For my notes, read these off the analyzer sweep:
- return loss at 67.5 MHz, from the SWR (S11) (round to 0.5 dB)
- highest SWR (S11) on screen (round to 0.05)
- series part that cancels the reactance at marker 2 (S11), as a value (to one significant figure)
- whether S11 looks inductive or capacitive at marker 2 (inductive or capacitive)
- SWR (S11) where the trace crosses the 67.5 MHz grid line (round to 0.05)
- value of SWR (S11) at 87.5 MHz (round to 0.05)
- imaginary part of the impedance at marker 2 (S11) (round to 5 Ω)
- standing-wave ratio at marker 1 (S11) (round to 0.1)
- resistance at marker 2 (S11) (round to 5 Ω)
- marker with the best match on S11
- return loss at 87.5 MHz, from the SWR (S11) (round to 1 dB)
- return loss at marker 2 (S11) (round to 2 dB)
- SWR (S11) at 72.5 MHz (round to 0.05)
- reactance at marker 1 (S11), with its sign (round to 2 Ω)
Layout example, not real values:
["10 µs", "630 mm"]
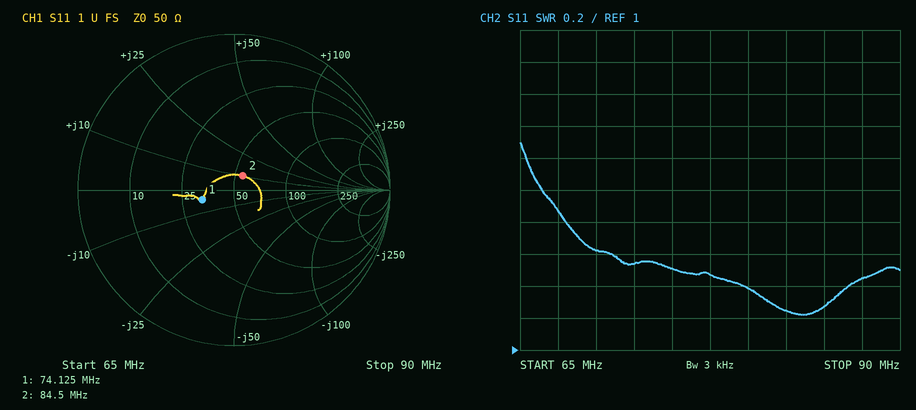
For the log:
["10.5 dB", "2.30", "200 pF", "inductive", "1.85", "1.45", "+10 Ω", "1.5", "55 Ω", "marker 2", "15 dB", "20 dB", "1.55", "-4 Ω"]
